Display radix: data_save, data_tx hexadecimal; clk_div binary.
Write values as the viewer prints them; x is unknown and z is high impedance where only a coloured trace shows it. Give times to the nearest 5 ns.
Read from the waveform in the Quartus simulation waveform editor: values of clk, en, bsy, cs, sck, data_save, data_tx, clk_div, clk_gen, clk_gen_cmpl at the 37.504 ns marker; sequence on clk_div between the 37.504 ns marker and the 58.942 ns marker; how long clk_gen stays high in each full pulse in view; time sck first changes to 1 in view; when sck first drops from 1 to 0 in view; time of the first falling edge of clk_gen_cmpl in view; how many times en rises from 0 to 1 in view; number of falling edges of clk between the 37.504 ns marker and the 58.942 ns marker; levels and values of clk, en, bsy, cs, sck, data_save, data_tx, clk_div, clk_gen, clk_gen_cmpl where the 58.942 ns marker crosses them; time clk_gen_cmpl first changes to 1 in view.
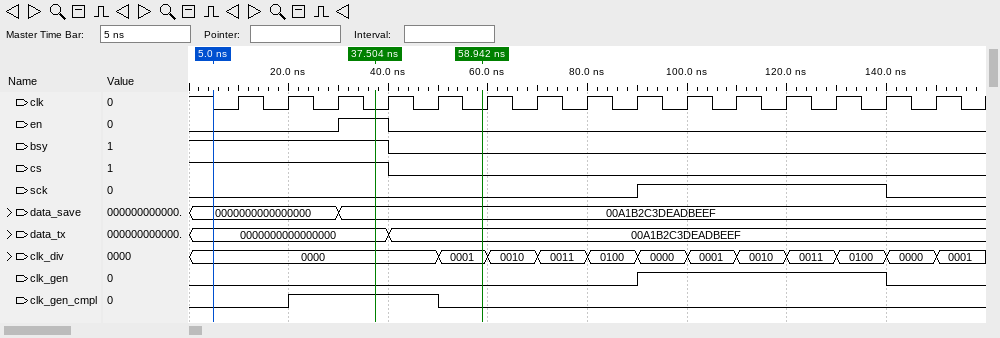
clk=0, en=1, bsy=1, cs=1, sck=0, data_save=00A1B2C3DEADBEEF, data_tx=0000000000000000, clk_div=0000, clk_gen=0, clk_gen_cmpl=1
0000, 0001
50 ns
90 ns
140 ns
50 ns
1
2
clk=0, en=0, bsy=0, cs=0, sck=0, data_save=00A1B2C3DEADBEEF, data_tx=00A1B2C3DEADBEEF, clk_div=0001, clk_gen=0, clk_gen_cmpl=0
20 ns
